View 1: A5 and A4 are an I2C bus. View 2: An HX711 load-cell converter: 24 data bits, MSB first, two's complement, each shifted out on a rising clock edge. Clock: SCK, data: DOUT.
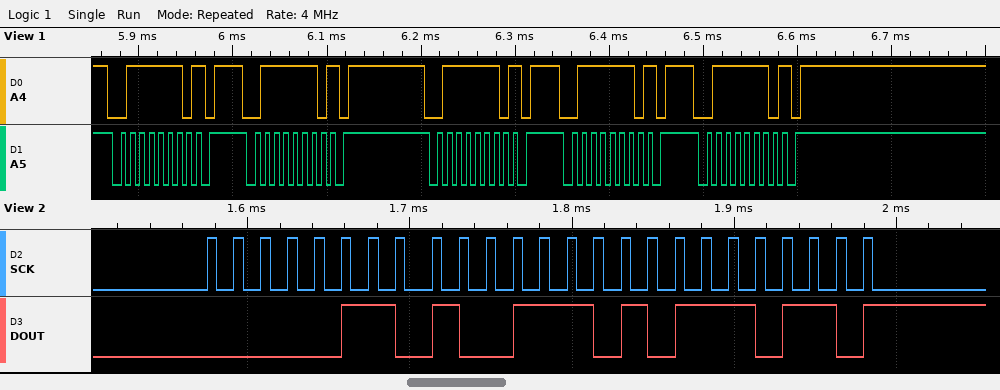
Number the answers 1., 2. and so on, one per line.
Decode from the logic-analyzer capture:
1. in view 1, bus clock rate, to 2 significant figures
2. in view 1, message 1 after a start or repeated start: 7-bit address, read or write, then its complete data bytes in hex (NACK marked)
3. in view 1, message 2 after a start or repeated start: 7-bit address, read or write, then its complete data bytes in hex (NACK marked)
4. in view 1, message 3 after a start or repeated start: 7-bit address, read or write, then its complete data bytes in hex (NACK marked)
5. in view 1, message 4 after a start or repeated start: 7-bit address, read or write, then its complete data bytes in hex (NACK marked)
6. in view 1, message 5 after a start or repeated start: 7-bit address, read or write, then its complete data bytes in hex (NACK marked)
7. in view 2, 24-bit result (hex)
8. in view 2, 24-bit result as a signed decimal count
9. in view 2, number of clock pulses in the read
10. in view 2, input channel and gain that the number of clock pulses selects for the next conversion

1. 100 kHz
2. 0x3F write NACK
3. 0x3F write NACK
4. 0x3F write NACK
5. 0x3F write NACK
6. 0x3F write NACK
7. 0x069D76
8. 433526
9. 25
10. channel A, gain 128
